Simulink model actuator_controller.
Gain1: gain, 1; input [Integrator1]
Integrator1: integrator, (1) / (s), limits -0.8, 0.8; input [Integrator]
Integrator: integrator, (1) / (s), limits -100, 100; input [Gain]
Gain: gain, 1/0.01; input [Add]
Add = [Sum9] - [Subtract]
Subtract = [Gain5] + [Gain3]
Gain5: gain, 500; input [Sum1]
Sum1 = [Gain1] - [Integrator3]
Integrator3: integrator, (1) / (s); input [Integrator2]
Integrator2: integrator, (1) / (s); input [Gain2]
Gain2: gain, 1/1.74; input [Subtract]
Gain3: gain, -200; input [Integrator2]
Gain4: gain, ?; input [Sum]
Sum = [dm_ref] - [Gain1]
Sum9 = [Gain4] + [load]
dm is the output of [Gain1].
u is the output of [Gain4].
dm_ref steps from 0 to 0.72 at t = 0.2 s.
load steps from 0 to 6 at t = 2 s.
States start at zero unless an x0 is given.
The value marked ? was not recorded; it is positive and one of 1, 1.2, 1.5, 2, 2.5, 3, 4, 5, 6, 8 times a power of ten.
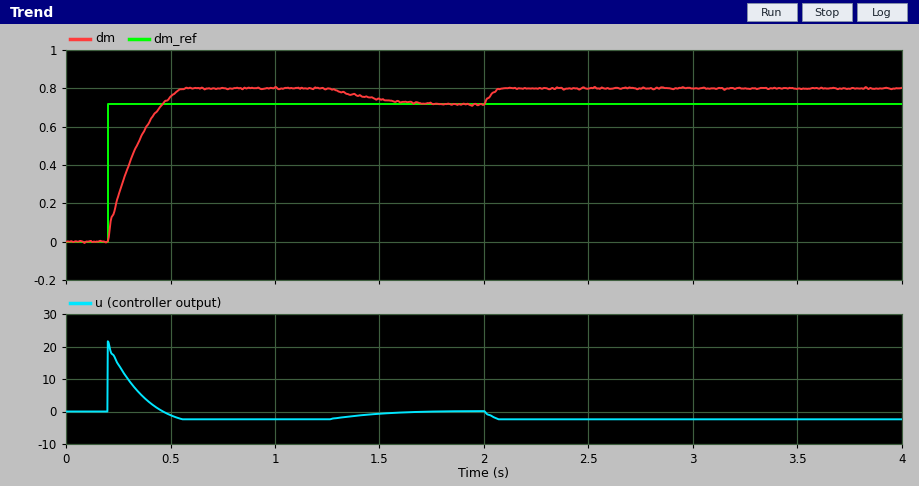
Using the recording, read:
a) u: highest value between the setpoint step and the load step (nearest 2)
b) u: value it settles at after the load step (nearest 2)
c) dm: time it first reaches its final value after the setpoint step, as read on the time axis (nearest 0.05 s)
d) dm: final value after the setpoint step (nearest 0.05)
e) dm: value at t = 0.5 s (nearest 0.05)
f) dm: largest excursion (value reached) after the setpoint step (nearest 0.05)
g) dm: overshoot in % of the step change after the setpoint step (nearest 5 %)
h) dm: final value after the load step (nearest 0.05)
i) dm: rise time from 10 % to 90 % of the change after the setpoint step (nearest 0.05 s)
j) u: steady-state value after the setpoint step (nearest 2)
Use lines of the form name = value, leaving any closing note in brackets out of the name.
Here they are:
u: highest value between the setpoint step and the load step = 22
u: value it settles at after the load step = -2
dm: time it first reaches its final value after the setpoint step, as read on the time axis = 0.45 s
dm: final value after the setpoint step = 0.70
dm: value at t = 0.5 s = 0.75
dm: largest excursion (value reached) after the setpoint step = 0.80
dm: overshoot in % of the step change after the setpoint step = 10 %
dm: final value after the load step = 0.80
dm: rise time from 10 % to 90 % of the change after the setpoint step = 0.20 s
u: steady-state value after the setpoint step = 0
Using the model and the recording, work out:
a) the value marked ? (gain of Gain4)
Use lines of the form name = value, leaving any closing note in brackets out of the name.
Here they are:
the value marked ? = 30
